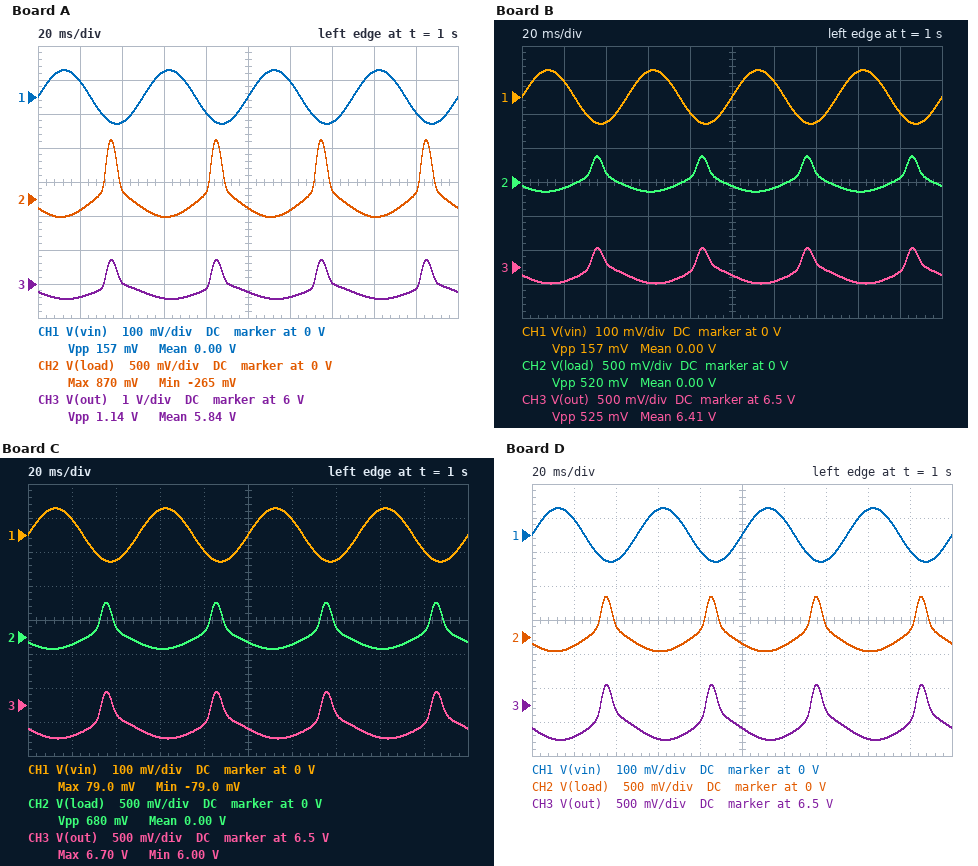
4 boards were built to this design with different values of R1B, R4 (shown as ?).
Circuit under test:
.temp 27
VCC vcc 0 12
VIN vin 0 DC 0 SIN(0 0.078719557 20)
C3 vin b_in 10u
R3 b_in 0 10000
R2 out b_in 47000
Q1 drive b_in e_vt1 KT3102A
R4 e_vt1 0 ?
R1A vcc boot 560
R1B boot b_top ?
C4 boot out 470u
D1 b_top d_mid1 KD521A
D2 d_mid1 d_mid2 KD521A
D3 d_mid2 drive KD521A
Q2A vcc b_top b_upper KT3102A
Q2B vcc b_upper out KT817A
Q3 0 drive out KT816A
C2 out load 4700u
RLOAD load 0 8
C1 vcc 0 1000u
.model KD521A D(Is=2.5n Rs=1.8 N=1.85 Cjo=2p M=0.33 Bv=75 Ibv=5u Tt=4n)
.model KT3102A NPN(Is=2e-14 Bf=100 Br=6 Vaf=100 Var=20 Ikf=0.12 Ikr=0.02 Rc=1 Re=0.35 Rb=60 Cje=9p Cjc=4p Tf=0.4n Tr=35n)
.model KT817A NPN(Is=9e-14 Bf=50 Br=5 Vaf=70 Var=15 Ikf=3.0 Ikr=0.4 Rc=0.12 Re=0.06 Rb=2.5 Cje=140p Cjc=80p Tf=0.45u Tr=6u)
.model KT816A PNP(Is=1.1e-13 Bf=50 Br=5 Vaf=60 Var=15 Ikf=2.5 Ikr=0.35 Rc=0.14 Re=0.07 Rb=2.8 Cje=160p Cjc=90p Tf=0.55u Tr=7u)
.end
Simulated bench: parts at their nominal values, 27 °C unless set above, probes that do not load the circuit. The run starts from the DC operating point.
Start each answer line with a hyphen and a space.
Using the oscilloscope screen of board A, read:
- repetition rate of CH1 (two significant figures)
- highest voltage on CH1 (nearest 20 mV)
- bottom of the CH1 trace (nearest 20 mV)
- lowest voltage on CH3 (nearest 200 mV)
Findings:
- 20 Hz
- 80 mV
- -80 mV
- 5.6 V
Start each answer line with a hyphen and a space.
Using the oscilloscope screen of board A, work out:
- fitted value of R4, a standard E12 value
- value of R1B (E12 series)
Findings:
- 180 Ω
- 3.9 kΩ
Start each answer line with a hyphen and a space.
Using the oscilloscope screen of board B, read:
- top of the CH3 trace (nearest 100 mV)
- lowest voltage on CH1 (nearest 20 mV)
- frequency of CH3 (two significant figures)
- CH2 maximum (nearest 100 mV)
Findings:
- 6.8 V
- -80 mV
- 20 Hz
- 400 mV
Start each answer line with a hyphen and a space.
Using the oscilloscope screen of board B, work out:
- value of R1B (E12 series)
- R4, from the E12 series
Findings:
- 3.9 kΩ
- 330 Ω
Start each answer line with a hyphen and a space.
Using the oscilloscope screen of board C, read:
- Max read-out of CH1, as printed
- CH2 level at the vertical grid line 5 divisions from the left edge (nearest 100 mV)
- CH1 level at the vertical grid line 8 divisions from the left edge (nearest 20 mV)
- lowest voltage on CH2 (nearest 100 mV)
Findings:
- 79.0 mV
- -100 mV
- 80 mV
- -200 mV
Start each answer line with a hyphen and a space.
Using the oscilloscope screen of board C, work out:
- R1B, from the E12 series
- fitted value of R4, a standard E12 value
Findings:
- 3.9 kΩ
- 270 Ω
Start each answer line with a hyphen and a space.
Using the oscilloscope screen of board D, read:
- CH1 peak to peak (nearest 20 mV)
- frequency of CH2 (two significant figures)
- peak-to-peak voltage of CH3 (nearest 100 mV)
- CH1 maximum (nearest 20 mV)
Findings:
- 160 mV
- 20 Hz
- 800 mV
- 80 mV
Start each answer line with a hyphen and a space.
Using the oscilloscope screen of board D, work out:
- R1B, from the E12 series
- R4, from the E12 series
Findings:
- 3.3 kΩ
- 220 Ω
